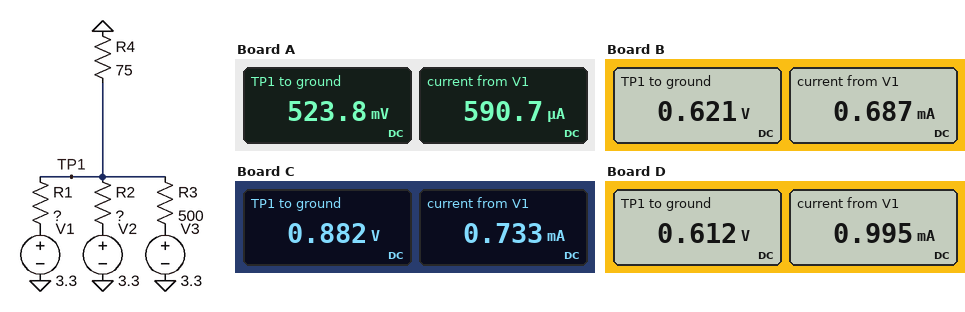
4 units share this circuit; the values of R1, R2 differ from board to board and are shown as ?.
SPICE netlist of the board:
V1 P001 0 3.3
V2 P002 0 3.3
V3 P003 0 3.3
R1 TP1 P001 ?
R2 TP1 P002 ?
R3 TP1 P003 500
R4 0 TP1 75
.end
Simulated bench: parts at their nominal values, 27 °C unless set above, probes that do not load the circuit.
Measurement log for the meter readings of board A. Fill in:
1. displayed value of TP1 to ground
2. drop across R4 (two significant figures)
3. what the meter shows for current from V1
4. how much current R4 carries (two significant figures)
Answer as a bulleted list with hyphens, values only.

- 523.8 mV
- 520 mV
- 590.7 µA
- 7.0 mA
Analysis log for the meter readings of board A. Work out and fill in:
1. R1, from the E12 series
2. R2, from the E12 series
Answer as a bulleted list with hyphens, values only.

- 4.7 kΩ
- 3.3 kΩ
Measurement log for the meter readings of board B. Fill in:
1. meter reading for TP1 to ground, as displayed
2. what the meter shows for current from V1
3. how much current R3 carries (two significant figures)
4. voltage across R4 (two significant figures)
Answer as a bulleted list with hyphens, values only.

- 0.621 V
- 0.687 mA
- 5.4 mA
- 620 mV
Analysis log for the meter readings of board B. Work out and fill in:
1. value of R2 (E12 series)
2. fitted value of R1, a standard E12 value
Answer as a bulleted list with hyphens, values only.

- 1.2 kΩ
- 3.9 kΩ
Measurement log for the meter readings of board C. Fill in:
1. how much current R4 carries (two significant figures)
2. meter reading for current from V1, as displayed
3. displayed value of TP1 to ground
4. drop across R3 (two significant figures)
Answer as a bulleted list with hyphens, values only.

- 12 mA
- 0.733 mA
- 0.882 V
- 2.4 V
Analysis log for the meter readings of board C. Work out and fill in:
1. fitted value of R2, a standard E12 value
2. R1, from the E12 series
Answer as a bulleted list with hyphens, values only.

- 390 Ω
- 3.3 kΩ
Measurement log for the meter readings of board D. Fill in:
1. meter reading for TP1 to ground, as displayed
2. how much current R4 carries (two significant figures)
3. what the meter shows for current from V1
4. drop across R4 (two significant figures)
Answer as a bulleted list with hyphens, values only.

- 0.612 V
- 8.2 mA
- 0.995 mA
- 610 mV
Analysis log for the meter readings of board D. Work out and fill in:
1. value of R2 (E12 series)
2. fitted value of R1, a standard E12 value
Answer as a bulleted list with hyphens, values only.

- 1.5 kΩ
- 2.7 kΩ
